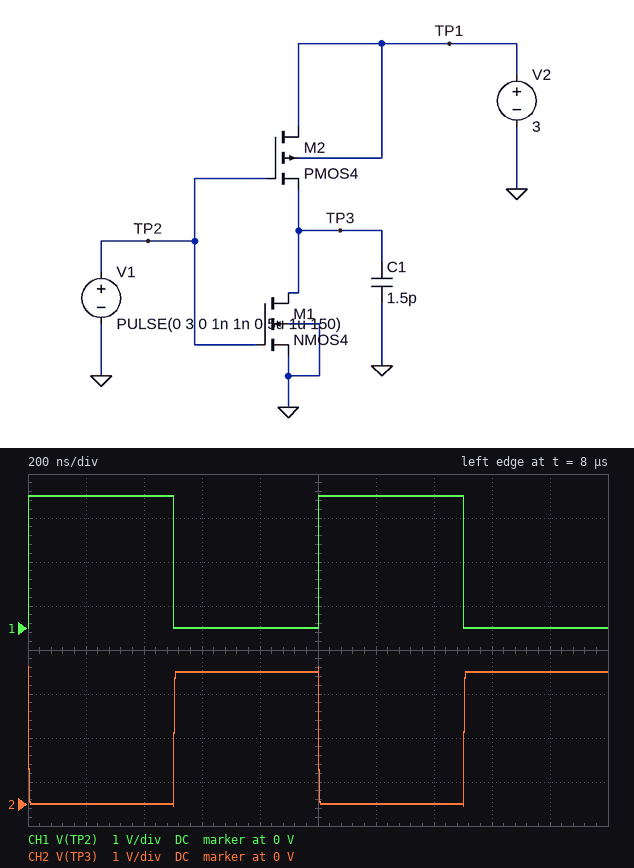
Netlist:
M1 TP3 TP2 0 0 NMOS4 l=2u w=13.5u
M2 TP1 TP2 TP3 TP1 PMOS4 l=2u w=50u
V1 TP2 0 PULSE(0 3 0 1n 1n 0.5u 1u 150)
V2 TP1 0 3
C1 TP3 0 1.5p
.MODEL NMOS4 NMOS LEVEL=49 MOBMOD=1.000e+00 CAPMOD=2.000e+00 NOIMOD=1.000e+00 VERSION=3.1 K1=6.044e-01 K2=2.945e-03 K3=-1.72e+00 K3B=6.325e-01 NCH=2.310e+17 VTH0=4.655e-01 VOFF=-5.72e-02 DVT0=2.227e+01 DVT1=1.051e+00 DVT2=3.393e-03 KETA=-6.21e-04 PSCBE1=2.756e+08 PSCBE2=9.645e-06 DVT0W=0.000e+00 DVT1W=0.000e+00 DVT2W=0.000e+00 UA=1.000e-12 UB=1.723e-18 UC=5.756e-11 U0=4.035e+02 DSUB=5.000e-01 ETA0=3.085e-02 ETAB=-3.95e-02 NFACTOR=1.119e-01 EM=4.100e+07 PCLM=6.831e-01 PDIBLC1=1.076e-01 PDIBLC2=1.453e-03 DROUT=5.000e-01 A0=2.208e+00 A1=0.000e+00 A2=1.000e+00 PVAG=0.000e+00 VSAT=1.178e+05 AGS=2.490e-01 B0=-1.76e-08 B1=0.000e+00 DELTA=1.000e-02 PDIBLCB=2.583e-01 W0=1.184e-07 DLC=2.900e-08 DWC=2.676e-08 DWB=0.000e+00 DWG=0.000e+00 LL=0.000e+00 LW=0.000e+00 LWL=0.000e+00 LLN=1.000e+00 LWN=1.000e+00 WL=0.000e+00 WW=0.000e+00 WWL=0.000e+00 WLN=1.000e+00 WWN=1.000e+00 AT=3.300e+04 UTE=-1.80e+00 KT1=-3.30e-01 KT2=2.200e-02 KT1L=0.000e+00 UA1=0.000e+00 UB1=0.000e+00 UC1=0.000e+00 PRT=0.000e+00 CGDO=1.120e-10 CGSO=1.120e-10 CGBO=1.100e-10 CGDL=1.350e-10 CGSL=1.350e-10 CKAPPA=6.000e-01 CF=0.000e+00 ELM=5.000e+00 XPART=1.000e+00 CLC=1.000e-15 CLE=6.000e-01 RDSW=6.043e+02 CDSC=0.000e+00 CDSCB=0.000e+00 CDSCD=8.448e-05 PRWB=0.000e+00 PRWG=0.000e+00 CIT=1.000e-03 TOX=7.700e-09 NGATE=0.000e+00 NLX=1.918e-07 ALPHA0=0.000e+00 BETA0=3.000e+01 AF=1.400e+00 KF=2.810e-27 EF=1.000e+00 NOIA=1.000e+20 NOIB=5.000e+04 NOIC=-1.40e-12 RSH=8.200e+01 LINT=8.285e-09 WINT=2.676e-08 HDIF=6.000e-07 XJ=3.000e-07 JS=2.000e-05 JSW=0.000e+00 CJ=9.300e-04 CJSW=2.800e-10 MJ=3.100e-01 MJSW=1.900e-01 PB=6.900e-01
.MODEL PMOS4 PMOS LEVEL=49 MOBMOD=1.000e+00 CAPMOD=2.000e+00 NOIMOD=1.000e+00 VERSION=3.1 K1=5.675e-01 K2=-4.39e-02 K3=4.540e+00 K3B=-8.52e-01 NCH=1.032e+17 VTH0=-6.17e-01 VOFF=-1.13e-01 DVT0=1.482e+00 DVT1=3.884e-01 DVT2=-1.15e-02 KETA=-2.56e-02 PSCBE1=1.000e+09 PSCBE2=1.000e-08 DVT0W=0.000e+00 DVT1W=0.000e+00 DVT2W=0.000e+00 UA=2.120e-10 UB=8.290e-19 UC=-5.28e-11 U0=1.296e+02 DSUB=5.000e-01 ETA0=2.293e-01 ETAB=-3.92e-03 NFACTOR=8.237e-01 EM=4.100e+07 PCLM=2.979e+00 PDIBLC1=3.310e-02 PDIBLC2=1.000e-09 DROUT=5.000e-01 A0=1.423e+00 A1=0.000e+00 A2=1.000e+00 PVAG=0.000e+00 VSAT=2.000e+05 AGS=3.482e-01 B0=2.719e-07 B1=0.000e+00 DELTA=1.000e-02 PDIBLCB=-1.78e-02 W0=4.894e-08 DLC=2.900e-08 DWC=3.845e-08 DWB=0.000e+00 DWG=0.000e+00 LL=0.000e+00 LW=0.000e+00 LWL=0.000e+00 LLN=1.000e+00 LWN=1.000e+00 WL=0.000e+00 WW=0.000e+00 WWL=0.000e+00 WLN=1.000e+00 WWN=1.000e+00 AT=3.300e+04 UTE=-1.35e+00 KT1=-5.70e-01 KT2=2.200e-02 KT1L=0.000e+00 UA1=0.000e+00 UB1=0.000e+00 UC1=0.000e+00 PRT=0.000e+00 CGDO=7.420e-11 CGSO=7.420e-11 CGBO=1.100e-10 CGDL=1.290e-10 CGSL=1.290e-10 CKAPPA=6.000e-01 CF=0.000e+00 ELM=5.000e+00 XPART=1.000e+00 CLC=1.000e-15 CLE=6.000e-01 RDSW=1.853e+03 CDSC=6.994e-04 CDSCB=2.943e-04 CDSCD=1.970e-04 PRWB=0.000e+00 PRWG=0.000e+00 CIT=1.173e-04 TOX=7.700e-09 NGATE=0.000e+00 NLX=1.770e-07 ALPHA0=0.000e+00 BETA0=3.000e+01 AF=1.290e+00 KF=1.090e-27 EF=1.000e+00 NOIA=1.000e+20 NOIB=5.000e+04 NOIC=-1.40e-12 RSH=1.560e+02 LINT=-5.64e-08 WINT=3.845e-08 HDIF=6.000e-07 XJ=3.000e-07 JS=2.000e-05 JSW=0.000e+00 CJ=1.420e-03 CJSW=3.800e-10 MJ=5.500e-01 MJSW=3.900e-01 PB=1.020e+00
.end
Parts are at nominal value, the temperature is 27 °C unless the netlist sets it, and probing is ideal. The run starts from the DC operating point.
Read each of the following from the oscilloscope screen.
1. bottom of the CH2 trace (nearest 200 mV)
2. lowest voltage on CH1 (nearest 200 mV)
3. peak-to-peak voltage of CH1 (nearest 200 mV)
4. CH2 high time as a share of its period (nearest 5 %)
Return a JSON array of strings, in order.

["0 V", "0 V", "3.0 V", "50 %"]
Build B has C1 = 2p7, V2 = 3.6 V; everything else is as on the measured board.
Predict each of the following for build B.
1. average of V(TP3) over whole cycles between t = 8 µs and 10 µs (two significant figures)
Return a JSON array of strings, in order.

["1.8 V"]
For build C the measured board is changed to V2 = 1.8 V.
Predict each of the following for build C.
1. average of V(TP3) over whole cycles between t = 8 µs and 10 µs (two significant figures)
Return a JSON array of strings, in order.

["890 mV"]
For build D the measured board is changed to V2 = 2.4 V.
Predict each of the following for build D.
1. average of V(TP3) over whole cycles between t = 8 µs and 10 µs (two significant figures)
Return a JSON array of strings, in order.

["1.2 V"]
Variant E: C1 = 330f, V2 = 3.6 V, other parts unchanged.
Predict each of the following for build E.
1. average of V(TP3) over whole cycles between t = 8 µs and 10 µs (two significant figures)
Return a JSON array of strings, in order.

["1.8 V"]
